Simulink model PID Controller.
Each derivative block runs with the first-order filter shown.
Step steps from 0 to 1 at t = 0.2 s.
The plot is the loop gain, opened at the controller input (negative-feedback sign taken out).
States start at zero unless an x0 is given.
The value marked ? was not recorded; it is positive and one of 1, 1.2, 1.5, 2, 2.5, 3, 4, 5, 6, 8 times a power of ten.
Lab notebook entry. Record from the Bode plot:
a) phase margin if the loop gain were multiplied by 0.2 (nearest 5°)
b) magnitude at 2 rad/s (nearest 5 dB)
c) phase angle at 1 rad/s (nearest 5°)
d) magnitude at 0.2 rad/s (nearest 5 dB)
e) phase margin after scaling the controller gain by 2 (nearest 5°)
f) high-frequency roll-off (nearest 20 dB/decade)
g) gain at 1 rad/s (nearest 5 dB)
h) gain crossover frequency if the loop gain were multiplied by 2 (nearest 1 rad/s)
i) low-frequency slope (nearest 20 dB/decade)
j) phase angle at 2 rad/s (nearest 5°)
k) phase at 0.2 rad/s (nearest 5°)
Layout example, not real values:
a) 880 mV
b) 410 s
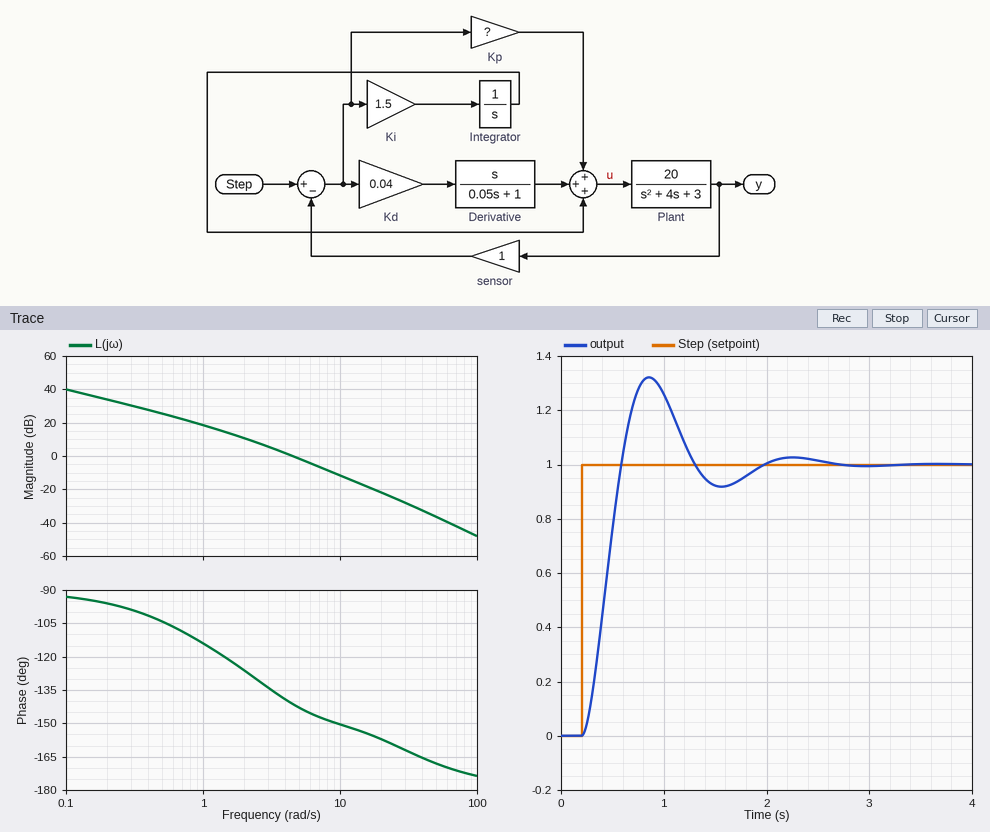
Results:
a) 60°
b) 10 dB
c) -115°
d) 35 dB
e) 35°
f) -40 dB/decade
g) 20 dB
h) 7 rad/s
i) -20 dB/decade
j) -125°
k) -95°
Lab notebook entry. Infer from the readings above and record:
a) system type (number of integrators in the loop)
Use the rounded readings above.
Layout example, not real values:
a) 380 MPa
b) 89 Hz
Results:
a) 1
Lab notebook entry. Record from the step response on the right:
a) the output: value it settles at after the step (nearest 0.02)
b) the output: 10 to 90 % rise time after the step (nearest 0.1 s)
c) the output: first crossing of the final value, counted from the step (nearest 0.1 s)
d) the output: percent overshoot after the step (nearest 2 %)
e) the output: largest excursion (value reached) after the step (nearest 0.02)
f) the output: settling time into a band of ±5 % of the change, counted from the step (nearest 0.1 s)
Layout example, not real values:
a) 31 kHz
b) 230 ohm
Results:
a) 1.00
b) 0.3 s
c) 0.4 s
d) 32 %
e) 1.32
f) 1.6 s
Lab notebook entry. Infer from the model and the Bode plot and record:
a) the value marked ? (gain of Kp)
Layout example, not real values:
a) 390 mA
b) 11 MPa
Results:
a) 1.2
